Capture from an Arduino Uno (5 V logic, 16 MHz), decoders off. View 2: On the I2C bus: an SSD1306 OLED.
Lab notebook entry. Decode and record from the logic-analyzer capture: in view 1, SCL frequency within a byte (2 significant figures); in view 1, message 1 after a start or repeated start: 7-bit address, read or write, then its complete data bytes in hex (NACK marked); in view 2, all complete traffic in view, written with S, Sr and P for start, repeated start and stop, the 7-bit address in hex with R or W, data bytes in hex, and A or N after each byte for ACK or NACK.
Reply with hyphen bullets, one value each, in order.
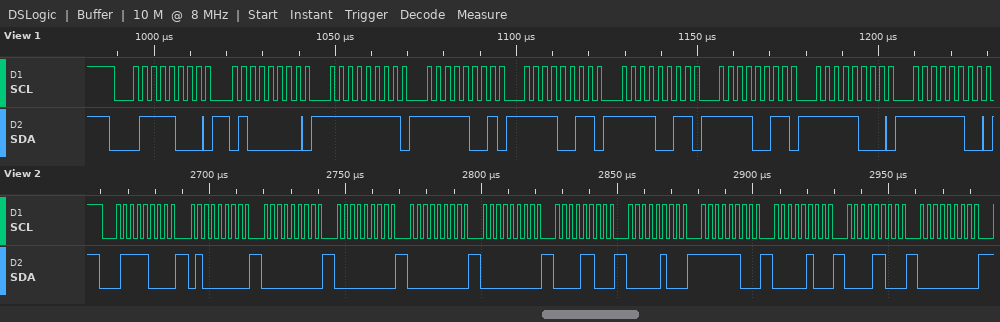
- 400 kHz
- 0x3C write: 40 FF F9 F3 F3 F3 F8 FC
- S 3CW A 40 A 00 A 00 A 00 A 00 A 0C A 04 A FC A 04 A 0C A 00 A
